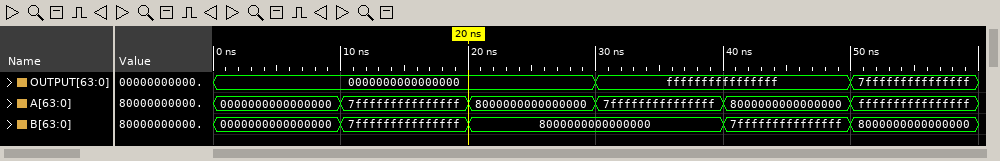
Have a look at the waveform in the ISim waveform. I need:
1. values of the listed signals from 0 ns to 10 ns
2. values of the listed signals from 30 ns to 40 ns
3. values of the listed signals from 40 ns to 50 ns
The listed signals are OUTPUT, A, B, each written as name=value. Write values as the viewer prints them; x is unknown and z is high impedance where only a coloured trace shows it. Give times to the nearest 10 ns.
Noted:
OUTPUT=0000000000000000, A=0000000000000000, B=0000000000000000
OUTPUT=ffffffffffffffff, A=7fffffffffffffff, B=8000000000000000
OUTPUT=ffffffffffffffff, A=8000000000000000, B=7fffffffffffffff
